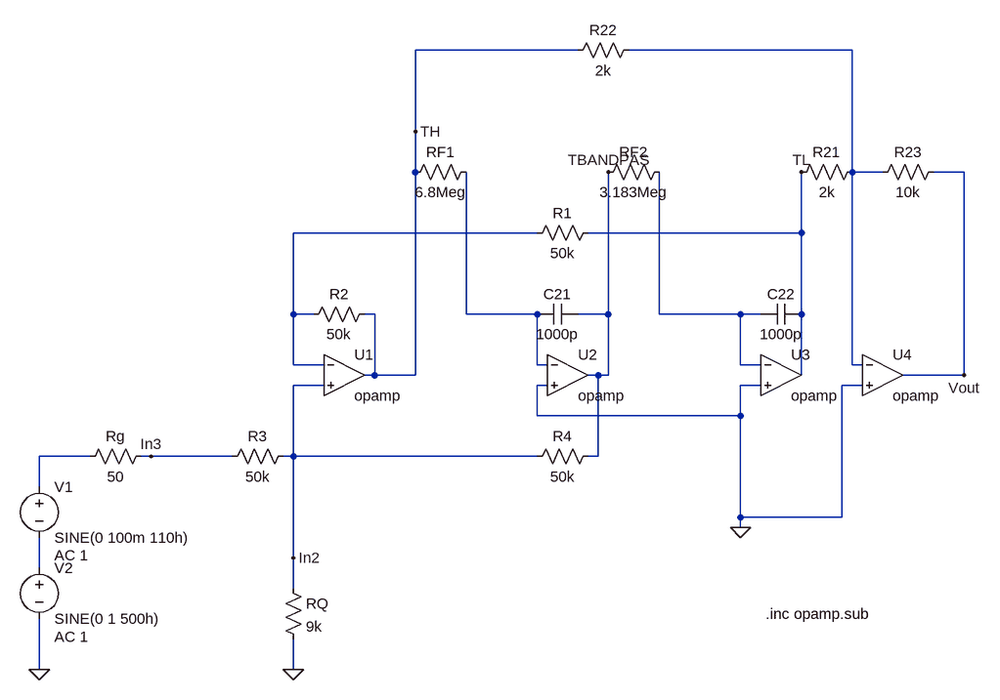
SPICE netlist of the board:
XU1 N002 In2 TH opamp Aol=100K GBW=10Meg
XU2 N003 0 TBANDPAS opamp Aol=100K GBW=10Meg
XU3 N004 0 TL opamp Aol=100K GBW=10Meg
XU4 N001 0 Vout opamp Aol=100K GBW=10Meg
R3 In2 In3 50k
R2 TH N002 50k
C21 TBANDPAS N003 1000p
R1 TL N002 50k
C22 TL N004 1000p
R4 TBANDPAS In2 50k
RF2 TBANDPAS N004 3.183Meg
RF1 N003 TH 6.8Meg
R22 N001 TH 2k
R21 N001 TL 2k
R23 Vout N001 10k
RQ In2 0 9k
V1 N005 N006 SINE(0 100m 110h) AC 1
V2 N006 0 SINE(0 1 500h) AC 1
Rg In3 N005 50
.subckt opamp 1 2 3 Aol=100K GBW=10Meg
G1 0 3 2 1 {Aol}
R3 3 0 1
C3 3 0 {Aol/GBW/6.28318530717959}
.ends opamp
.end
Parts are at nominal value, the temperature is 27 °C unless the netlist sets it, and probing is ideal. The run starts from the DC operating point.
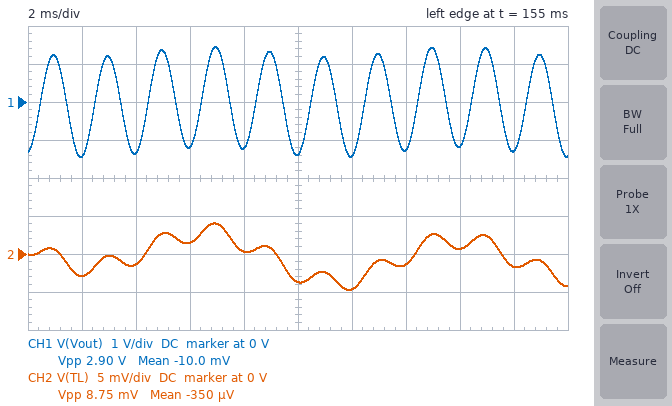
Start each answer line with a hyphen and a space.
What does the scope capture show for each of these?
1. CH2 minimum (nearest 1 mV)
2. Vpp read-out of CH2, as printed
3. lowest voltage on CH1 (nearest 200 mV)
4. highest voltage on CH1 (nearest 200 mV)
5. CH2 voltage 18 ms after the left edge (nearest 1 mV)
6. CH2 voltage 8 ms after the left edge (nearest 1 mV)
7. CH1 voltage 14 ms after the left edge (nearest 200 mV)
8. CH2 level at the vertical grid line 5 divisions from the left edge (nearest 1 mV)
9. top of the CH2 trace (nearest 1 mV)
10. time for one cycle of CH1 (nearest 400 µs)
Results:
- -5 mV
- 8.75 mV
- -1.4 V
- 1.4 V
- -2 mV
- 0 V
- -1.2 V
- -4 mV
- 4 mV
- 2.0 ms
